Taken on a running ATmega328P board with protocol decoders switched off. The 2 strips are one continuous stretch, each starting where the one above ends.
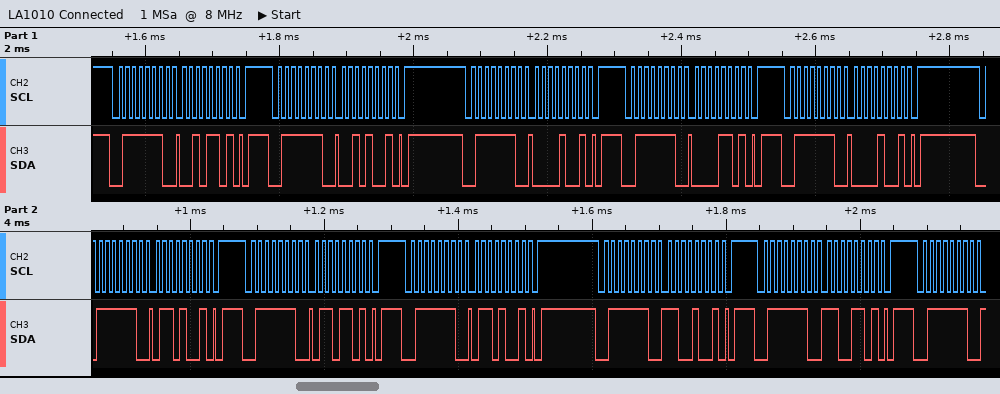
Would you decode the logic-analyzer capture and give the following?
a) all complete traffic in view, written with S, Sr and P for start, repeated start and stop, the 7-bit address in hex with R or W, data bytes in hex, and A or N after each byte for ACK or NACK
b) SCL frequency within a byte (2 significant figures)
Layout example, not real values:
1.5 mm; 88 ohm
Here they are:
S 3FW A 2D A P S 3FW A 29 A P S 3FW A 09 A P S 3FW A 0D A P S 3FW A 09 A P S 3FW A 69 A P S 3FW A 6D A P S 3FW A 69 A P S 3FW A C9 A P S 3FW A CD A P S 3FW A; 100 kHz
